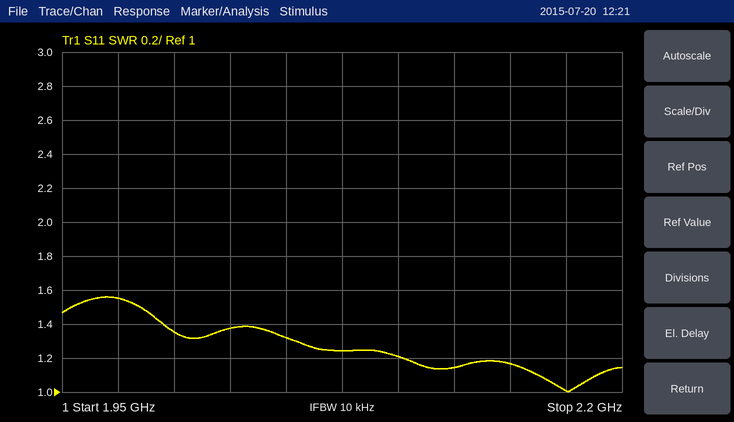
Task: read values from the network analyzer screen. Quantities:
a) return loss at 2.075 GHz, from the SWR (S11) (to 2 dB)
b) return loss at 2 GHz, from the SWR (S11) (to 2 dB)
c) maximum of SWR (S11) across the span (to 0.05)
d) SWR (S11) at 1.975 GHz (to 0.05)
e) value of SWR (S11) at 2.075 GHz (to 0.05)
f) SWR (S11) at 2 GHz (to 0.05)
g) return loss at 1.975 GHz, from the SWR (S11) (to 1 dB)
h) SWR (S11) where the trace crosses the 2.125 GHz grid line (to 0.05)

20 dB
16 dB
1.55
1.55
1.25
1.35
13 dB
1.15
